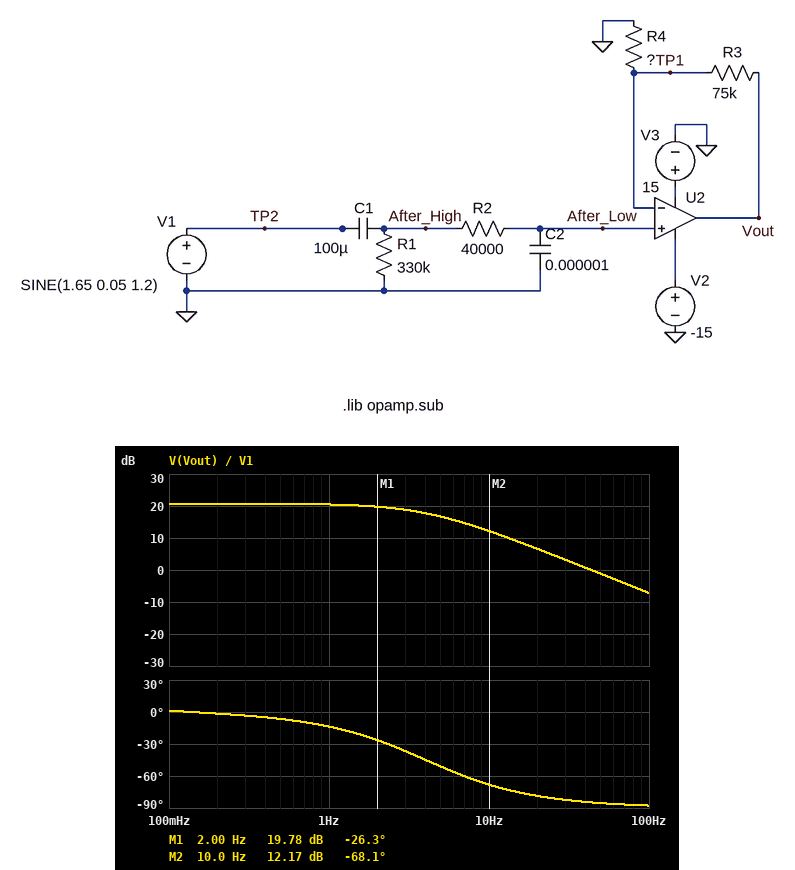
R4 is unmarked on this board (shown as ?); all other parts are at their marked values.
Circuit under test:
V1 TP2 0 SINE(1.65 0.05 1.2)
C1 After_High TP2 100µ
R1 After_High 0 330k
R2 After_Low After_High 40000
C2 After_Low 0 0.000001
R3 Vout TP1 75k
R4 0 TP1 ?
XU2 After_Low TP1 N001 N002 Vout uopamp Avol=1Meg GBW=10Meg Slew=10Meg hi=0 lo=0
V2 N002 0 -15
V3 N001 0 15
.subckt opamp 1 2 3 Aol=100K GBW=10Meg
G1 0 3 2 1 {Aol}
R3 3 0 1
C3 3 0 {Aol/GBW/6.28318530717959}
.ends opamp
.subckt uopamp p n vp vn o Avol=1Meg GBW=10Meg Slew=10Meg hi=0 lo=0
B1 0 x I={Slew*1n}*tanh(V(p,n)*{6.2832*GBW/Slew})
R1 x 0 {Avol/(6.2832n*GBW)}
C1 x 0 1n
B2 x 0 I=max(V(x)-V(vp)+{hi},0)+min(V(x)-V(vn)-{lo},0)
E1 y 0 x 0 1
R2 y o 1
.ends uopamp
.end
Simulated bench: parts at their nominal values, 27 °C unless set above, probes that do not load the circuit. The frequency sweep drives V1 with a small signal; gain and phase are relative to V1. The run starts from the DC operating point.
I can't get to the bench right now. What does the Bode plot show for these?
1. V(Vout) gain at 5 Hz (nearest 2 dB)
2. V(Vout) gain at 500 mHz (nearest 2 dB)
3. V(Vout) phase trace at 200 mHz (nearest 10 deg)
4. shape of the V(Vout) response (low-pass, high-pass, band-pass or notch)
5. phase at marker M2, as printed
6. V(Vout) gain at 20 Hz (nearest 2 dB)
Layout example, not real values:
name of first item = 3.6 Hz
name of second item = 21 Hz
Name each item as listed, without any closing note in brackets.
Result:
V(Vout) gain at 5 Hz = 16 dB
V(Vout) gain at 500 mHz = 20 dB
V(Vout) phase trace at 200 mHz = 0 deg
shape of the V(Vout) response = low-pass
phase at marker M2, as printed = -68.1 deg
V(Vout) gain at 20 Hz = 6 dB
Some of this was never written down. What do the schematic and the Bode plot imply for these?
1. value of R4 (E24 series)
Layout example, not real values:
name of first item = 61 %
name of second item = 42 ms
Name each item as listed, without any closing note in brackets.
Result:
value of R4 = 7.5 kΩ
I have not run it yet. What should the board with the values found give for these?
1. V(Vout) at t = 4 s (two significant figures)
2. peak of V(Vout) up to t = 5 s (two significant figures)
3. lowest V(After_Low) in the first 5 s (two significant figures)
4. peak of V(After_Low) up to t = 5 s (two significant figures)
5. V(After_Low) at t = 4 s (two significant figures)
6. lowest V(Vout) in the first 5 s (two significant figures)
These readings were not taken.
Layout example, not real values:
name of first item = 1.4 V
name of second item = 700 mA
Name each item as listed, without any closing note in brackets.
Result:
V(Vout) at t = 4 s = -520 mV
peak of V(Vout) up to t = 5 s = 520 mV
lowest V(After_Low) in the first 5 s = -48 mV
peak of V(After_Low) up to t = 5 s = 47 mV
V(After_Low) at t = 4 s = -48 mV
lowest V(Vout) in the first 5 s = -520 mV
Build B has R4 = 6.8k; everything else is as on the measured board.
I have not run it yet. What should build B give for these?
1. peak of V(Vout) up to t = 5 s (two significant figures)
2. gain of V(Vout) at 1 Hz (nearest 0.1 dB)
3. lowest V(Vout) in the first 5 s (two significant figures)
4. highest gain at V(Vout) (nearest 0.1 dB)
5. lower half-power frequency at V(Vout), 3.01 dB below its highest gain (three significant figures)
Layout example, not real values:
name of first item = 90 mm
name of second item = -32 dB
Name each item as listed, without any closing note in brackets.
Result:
peak of V(Vout) up to t = 5 s = 570 mV
gain of V(Vout) at 1 Hz = 21.3 dB
lowest V(Vout) in the first 5 s = -570 mV
highest gain at V(Vout) = 21.5 dB
lower half-power frequency at V(Vout), 3.01 dB below its highest gain = 4.76 mHz
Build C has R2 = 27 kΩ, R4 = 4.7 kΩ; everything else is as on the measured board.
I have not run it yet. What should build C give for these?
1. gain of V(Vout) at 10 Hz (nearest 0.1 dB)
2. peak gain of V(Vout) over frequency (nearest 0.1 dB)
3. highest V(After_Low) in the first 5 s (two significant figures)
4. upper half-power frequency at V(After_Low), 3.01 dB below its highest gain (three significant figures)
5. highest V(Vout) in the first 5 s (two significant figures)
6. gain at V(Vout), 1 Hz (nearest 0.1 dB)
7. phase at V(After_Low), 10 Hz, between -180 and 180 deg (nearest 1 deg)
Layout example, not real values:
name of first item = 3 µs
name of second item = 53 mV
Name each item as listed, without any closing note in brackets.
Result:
gain of V(Vout) at 10 Hz = 18.7 dB
peak gain of V(Vout) over frequency = 24.5 dB
highest V(After_Low) in the first 5 s = 48 mV
upper half-power frequency at V(After_Low), 3.01 dB below its highest gain = 5.96 Hz
highest V(Vout) in the first 5 s = 820 mV
gain at V(Vout), 1 Hz = 24.4 dB
phase at V(After_Low), 10 Hz, between -180 and 180 deg = -59 deg
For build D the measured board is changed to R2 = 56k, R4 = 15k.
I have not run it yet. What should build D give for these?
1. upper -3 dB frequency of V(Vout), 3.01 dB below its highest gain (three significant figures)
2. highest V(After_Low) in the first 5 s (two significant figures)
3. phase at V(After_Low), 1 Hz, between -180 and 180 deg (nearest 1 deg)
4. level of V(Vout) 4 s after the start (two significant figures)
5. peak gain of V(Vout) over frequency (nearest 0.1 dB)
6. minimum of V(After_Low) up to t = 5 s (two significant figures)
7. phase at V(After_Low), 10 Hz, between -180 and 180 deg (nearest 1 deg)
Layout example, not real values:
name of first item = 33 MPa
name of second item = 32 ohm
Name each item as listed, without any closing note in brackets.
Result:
upper -3 dB frequency of V(Vout), 3.01 dB below its highest gain = 2.88 Hz
highest V(After_Low) in the first 5 s = 46 mV
phase at V(After_Low), 1 Hz, between -180 and 180 deg = -19 deg
level of V(Vout) 4 s after the start = -270 mV
peak gain of V(Vout) over frequency = 15.5 dB
minimum of V(After_Low) up to t = 5 s = -46 mV
phase at V(After_Low), 10 Hz, between -180 and 180 deg = -74 deg
